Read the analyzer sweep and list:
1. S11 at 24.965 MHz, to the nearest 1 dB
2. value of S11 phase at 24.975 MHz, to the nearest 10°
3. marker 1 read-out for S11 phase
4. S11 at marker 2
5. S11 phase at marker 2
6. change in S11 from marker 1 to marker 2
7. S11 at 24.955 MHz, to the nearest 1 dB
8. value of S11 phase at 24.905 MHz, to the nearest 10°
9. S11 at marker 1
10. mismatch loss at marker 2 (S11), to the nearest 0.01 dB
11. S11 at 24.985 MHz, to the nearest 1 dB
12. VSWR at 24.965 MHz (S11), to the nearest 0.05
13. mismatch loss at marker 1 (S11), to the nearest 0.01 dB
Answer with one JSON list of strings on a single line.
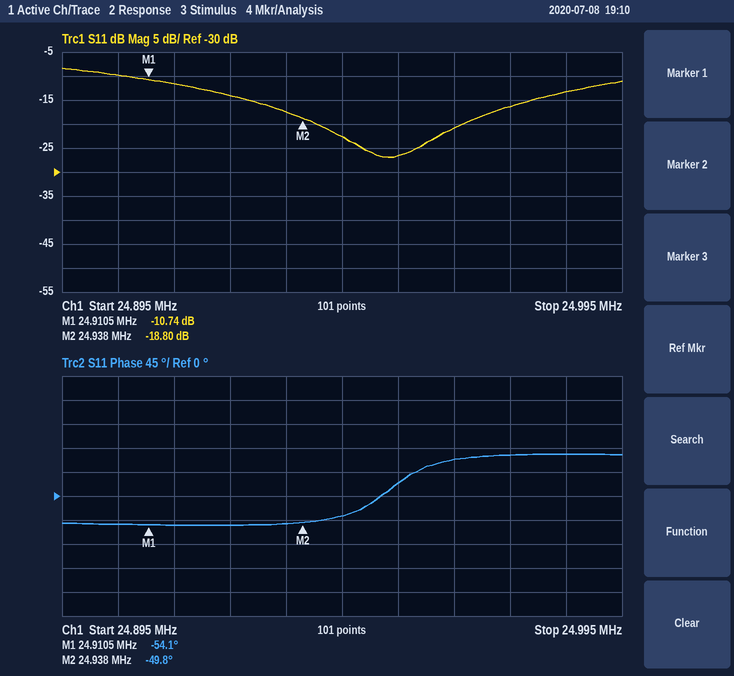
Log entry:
["-21 dB", "80°", "-54.1°", "-18.80 dB", "-49.8°", "-8.06 dB", "-27 dB", "-50°", "-10.74 dB", "0.06 dB", "-13 dB", "1.20", "0.38 dB"]
